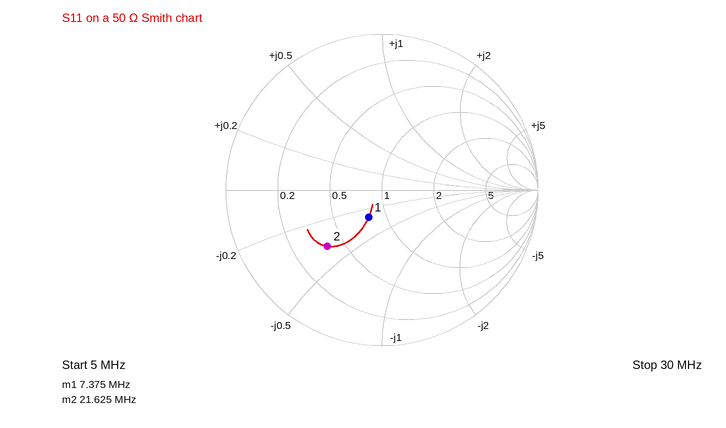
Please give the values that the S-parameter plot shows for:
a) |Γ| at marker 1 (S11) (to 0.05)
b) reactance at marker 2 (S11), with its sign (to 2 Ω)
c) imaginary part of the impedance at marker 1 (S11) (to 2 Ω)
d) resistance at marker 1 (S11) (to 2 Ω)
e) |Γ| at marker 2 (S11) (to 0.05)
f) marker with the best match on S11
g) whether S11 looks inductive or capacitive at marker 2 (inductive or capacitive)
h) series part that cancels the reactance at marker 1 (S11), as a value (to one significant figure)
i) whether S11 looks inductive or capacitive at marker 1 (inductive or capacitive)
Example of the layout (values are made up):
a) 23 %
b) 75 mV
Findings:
a) 0.20
b) -18 Ω
c) -14 Ω
d) 40 Ω
e) 0.50
f) marker 1
g) capacitive
h) 300 nH
i) capacitive
